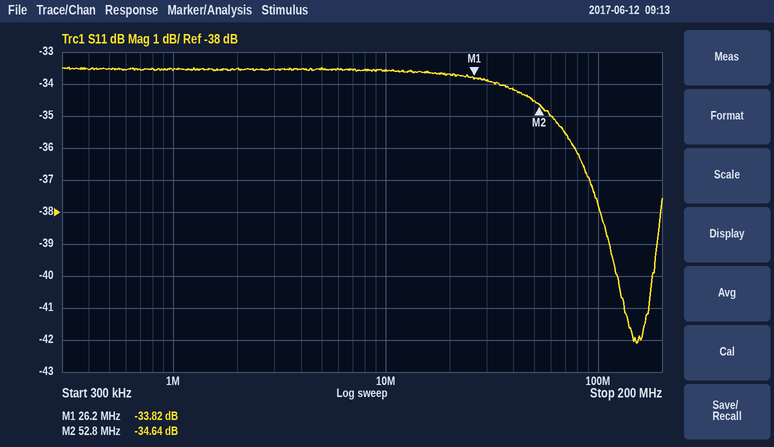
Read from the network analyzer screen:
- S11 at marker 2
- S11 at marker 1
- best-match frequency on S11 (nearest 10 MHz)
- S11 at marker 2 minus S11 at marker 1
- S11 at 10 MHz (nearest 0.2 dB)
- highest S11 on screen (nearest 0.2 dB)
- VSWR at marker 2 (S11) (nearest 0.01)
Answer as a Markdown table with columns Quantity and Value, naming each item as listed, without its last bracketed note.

| Quantity | Value |
|---|---|
| S11 at marker 2 | -34.64 dB |
| S11 at marker 1 | -33.82 dB |
| best-match frequency on S11 | 150 MHz |
| S11 at marker 2 minus S11 at marker 1 | -0.82 dB |
| S11 at 10 MHz | -33.6 dB |
| highest S11 on screen | -33.4 dB |
| VSWR at marker 2 (S11) | 1.04 |
